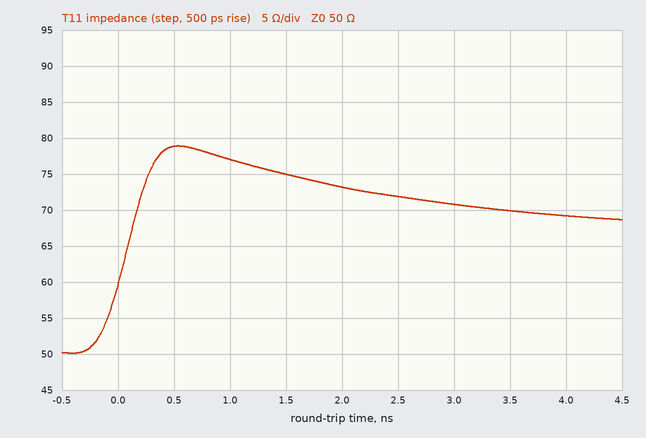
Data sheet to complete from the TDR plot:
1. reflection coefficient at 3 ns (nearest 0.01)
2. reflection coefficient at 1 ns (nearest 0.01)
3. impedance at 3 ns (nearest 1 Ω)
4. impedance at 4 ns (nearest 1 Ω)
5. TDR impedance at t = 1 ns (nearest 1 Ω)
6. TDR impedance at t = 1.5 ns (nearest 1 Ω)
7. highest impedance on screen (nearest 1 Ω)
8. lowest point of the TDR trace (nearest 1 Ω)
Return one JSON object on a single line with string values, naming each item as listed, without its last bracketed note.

{"reflection coefficient at 3 ns": "+0.17", "reflection coefficient at 1 ns": "+0.21", "impedance at 3 ns": "71 Ω", "impedance at 4 ns": "69 Ω", "TDR impedance at t = 1 ns": "77 Ω", "TDR impedance at t = 1.5 ns": "75 Ω", "highest impedance on screen": "79 Ω", "lowest point of the TDR trace": "50 Ω"}
